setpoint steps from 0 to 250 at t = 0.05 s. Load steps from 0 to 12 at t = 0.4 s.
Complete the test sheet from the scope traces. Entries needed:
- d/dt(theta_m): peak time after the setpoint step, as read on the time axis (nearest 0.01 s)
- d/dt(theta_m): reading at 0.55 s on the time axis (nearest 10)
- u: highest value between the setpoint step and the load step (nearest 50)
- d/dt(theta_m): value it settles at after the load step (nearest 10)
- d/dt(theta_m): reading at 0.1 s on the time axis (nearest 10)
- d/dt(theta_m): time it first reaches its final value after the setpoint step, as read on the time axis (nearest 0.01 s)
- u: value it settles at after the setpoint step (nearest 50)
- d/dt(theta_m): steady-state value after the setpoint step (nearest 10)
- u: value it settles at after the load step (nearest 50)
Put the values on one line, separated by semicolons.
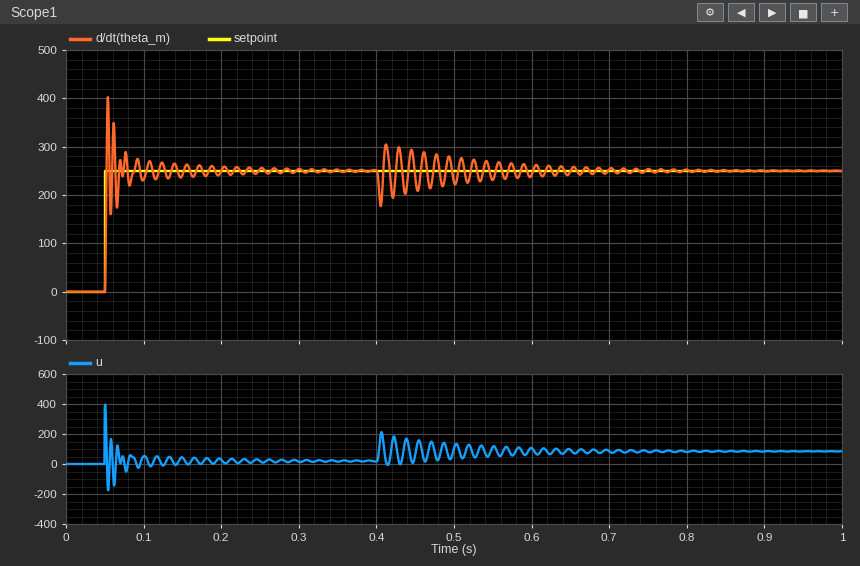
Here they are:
0.05 s; 230; 400; 250; 230; 0.05 s; 0; 250; 100
